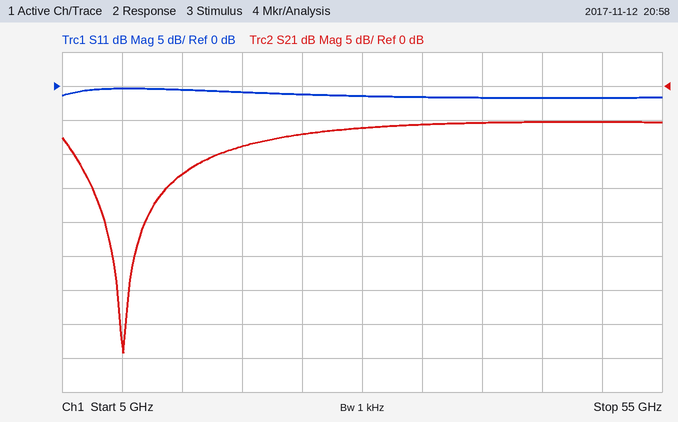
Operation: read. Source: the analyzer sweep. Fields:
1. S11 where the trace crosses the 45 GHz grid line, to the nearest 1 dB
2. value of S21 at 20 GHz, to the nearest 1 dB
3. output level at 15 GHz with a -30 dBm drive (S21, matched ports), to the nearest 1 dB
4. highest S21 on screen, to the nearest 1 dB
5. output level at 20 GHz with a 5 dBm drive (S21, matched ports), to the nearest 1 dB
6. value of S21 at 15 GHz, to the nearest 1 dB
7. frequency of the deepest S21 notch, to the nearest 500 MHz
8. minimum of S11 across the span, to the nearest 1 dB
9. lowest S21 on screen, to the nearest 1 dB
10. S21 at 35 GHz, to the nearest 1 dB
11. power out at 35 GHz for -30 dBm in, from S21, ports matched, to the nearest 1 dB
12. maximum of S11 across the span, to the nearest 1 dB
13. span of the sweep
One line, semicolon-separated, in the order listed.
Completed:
-2 dB; -9 dB; -43 dBm; -5 dB; -4 dBm; -13 dB; 10.0 GHz; -2 dB; -39 dB; -6 dB; -36 dBm; 0 dB; 50 GHz
